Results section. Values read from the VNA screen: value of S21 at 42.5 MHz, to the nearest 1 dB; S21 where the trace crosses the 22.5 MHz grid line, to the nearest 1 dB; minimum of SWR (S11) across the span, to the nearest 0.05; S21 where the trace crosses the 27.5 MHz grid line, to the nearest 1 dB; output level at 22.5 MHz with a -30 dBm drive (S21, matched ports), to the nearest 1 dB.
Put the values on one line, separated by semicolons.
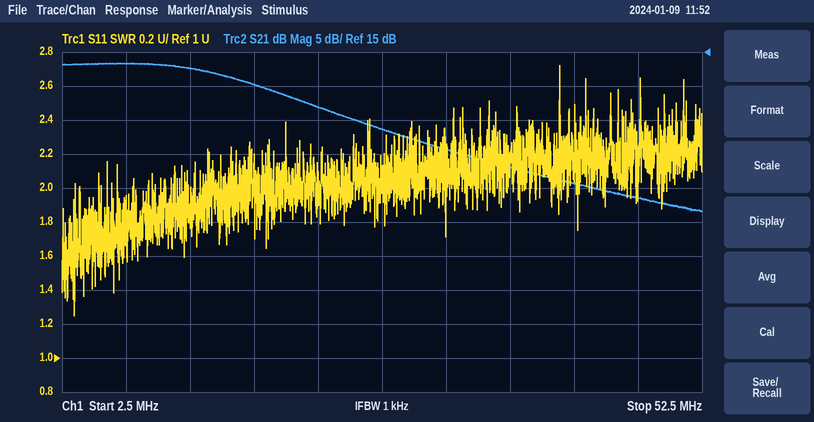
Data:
-4 dB; 7 dB; 1.25; 4 dB; -23 dBm
